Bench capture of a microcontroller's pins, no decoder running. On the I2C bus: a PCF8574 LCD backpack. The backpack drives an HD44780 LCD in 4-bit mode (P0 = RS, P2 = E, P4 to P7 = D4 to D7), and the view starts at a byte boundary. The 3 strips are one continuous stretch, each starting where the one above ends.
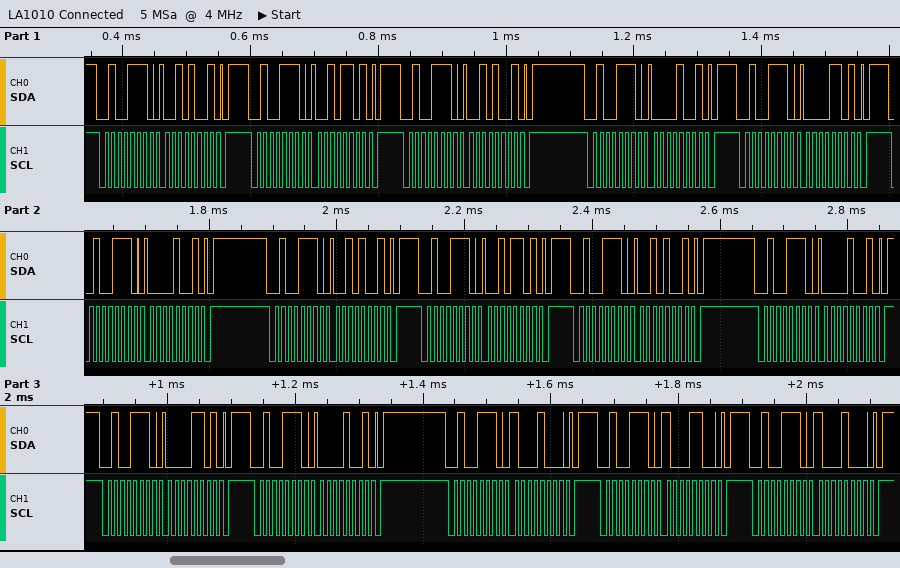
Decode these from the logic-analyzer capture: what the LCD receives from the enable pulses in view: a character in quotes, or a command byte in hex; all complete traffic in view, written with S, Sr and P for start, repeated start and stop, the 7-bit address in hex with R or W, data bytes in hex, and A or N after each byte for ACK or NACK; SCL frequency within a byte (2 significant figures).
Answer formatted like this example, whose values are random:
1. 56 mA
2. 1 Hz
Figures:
1. ' ' ' '
2. S 27W A 29 A P S 27W A 2D A P S 27W A 29 A P S 27W A 09 A P S 27W A 0D A P S 27W A 09 A P S 27W A 29 A P S 27W A 2D A P S 27W A 29 A P S 27W A 09 A P S 27W A 0D A P S 27W A 09 A P S 27W A 88 A P S 27W A 8C A P S 27W A 88 A P
3. 100 kHz
